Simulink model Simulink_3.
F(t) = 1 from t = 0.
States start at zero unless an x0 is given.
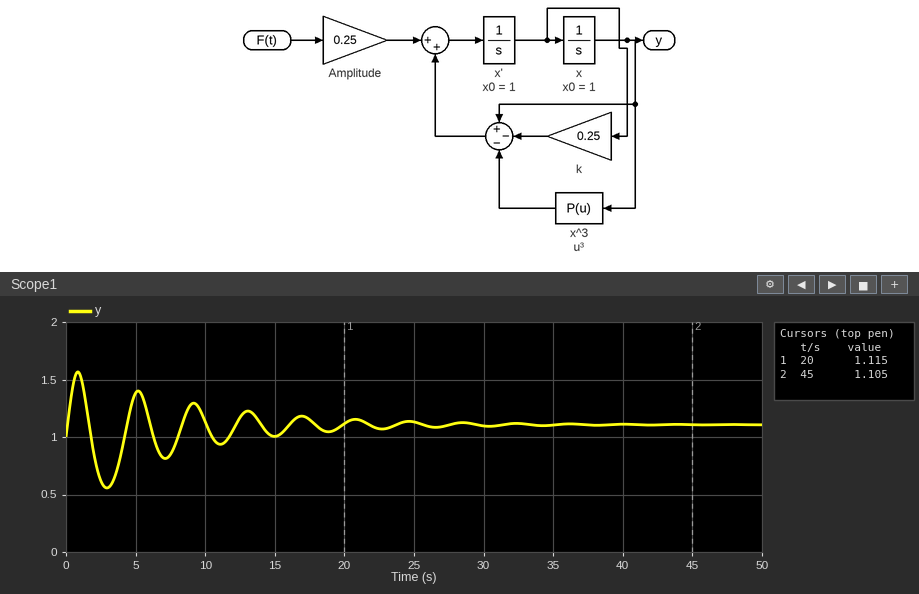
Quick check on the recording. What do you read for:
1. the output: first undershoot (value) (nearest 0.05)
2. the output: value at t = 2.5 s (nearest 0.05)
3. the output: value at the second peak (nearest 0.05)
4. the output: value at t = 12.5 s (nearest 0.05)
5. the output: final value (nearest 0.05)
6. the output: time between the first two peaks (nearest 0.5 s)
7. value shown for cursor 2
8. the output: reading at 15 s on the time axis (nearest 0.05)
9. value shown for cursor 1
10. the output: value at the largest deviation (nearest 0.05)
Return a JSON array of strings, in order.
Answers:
["0.55", "0.60", "1.40", "1.15", "1.10", "4.5 s", "1.105", "1.00", "1.115", "1.55"]
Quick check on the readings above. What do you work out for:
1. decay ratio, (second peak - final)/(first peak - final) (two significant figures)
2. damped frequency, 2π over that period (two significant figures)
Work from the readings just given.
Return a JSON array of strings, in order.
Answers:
["0.67", "1.4 rad/s"]
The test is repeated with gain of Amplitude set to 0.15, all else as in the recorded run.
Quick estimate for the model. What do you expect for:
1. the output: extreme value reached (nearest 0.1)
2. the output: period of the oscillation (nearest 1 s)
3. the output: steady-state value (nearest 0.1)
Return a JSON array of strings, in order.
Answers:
["1.5", "5 s", "1.1"]
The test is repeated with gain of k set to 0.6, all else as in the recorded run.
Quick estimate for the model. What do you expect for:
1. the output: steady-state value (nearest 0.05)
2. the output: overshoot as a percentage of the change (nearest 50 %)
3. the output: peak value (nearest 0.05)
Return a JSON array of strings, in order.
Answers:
["1.10", "350 %", "1.50"]
